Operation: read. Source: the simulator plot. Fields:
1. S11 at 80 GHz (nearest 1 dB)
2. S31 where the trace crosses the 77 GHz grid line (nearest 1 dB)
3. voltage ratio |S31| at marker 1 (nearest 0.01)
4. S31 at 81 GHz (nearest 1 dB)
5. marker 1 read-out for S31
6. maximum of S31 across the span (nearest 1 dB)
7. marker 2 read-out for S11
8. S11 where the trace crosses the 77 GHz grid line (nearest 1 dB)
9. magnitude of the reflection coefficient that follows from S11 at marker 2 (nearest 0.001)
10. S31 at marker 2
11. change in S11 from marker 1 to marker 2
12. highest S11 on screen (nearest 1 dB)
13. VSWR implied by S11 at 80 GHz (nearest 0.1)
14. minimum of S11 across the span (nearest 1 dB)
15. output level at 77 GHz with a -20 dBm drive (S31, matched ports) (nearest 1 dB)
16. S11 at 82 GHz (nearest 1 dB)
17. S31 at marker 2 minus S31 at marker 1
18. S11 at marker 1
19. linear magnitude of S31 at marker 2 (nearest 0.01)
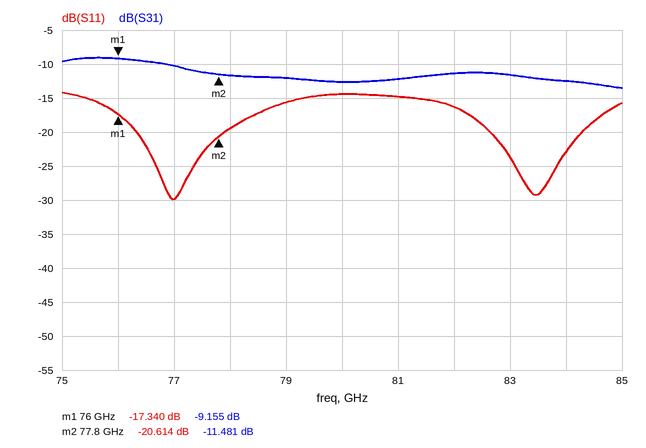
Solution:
-14 dB
-10 dB
0.35
-12 dB
-9.155 dB
-9 dB
-20.614 dB
-30 dB
0.093
-11.481 dB
-3.274 dB
-14 dB
1.5
-30 dB
-30 dBm
-16 dB
-2.326 dB
-17.340 dB
0.27
